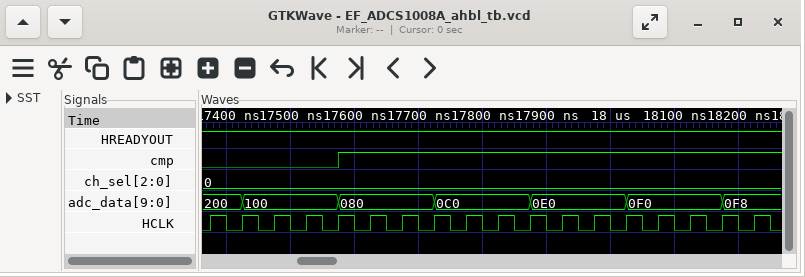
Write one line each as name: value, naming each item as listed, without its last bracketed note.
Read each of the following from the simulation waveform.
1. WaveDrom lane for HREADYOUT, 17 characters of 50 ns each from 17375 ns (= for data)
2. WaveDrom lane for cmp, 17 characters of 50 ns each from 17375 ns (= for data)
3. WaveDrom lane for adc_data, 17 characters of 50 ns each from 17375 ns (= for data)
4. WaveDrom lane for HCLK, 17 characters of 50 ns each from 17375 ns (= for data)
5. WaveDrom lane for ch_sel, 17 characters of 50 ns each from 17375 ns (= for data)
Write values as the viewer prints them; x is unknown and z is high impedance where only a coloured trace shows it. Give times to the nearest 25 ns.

WaveDrom lane for HREADYOUT, 17 characters of 50 ns each from 17375 ns: {name: 'HREADYOUT', wave: '1................'}
WaveDrom lane for cmp, 17 characters of 50 ns each from 17375 ns: {name: 'cmp', wave: '0...1............'}
WaveDrom lane for adc_data, 17 characters of 50 ns each from 17375 ns: {name: 'adc_data', wave: '==..=..=..=..=..=', data: '200 100 080 0C0 0E0 0F0 0F8'}
WaveDrom lane for HCLK, 17 characters of 50 ns each from 17375 ns: {name: 'HCLK', wave: 'p................'}
WaveDrom lane for ch_sel, 17 characters of 50 ns each from 17375 ns: {name: 'ch_sel', wave: '=................', data: '0'}
